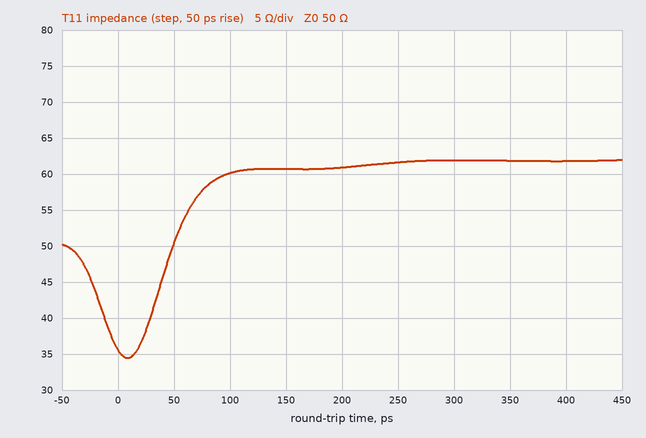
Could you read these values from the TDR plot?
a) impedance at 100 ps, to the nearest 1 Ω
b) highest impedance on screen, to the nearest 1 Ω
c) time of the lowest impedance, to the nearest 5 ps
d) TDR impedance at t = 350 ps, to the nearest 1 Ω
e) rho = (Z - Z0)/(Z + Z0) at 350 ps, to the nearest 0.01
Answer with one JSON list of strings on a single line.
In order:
["60 Ω", "62 Ω", "10 ps", "62 Ω", "+0.11"]
